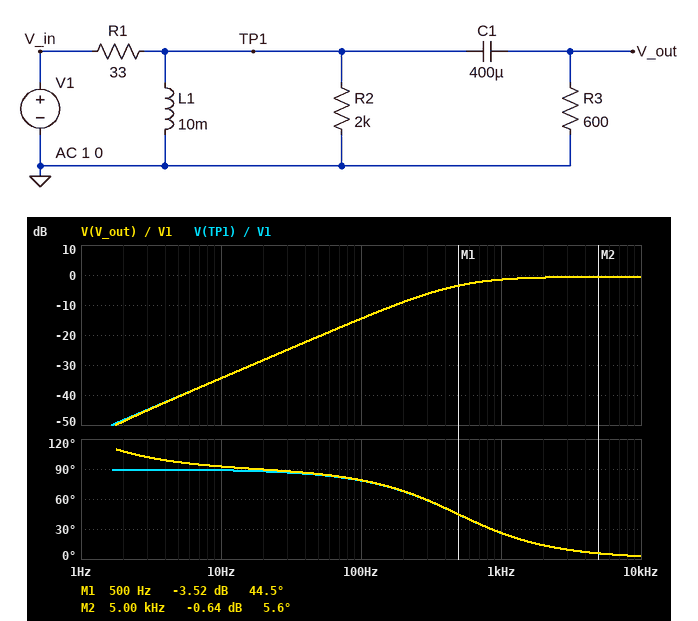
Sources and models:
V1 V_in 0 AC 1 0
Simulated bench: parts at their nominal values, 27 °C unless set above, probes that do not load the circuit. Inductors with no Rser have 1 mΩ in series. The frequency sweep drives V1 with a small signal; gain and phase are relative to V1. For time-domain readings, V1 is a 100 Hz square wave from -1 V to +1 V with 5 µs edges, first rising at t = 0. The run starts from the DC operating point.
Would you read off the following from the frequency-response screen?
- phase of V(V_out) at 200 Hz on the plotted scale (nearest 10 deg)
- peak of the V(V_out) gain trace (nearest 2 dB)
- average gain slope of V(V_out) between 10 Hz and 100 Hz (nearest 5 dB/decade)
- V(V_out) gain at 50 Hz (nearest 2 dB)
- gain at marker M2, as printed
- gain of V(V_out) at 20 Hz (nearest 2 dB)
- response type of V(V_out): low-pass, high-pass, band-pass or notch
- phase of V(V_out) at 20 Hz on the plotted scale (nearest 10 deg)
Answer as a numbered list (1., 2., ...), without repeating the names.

1. 70 deg
2. 0 dB
3. 20 dB/decade
4. -20 dB
5. -0.64 dB
6. -28 dB
7. high-pass
8. 90 deg
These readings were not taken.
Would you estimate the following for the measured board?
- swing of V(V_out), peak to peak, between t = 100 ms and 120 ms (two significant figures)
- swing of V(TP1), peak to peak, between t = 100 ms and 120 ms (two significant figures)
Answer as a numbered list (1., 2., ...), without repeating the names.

1. 3.7 V
2. 3.7 V
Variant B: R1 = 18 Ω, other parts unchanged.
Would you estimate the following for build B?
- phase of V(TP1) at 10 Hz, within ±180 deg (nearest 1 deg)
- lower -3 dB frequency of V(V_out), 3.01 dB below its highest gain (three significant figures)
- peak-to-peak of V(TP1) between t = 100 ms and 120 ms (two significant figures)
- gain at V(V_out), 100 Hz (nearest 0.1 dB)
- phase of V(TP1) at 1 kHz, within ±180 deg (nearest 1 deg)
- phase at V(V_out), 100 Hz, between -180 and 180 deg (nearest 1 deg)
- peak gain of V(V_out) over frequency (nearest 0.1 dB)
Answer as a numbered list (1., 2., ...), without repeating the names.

1. 88 deg
2. 276 Hz
3. 3.8 V
4. -9.7 dB
5. 15 deg
6. 70 deg
7. -0.3 dB
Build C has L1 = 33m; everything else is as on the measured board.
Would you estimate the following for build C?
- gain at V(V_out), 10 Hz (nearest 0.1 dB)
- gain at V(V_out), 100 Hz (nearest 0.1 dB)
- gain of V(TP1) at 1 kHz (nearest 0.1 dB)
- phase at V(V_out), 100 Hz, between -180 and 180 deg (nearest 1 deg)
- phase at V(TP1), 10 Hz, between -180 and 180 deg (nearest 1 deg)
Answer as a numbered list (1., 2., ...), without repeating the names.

1. -24.1 dB
2. -5.7 dB
3. -0.7 dB
4. 56 deg
5. 86 deg
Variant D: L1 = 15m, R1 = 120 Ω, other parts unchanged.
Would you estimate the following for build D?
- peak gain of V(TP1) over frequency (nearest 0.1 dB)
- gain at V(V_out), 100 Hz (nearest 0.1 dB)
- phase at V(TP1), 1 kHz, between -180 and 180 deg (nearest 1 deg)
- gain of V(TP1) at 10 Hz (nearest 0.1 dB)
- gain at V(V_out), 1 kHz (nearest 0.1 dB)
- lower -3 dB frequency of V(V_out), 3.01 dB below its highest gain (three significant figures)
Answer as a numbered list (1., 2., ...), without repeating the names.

1. -2.0 dB
2. -22.1 dB
3. 45 deg
4. -42.1 dB
5. -5.1 dB
6. 1.01 kHz
